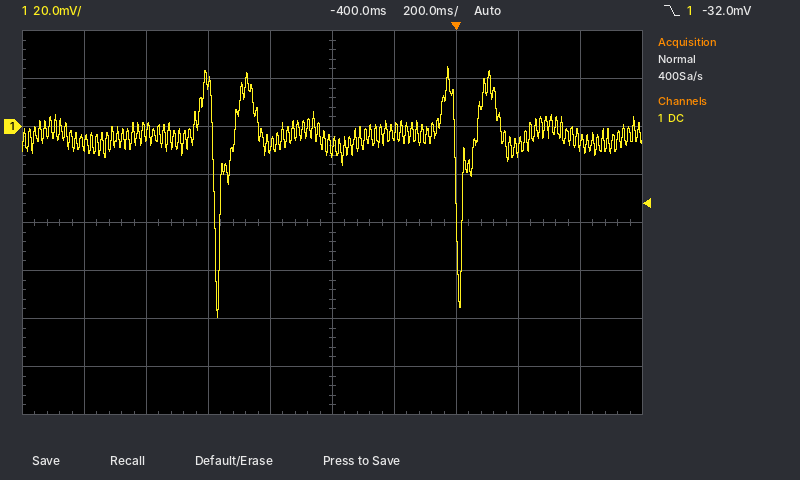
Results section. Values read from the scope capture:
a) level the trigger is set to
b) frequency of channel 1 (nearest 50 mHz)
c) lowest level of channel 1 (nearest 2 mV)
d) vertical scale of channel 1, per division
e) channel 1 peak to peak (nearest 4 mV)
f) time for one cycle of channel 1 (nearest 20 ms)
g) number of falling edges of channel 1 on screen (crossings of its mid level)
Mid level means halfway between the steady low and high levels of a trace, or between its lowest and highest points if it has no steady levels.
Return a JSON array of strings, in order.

["-32.0 mV", "1.30 Hz", "-80 mV", "20 mV", "104 mV", "780 ms", "2"]
